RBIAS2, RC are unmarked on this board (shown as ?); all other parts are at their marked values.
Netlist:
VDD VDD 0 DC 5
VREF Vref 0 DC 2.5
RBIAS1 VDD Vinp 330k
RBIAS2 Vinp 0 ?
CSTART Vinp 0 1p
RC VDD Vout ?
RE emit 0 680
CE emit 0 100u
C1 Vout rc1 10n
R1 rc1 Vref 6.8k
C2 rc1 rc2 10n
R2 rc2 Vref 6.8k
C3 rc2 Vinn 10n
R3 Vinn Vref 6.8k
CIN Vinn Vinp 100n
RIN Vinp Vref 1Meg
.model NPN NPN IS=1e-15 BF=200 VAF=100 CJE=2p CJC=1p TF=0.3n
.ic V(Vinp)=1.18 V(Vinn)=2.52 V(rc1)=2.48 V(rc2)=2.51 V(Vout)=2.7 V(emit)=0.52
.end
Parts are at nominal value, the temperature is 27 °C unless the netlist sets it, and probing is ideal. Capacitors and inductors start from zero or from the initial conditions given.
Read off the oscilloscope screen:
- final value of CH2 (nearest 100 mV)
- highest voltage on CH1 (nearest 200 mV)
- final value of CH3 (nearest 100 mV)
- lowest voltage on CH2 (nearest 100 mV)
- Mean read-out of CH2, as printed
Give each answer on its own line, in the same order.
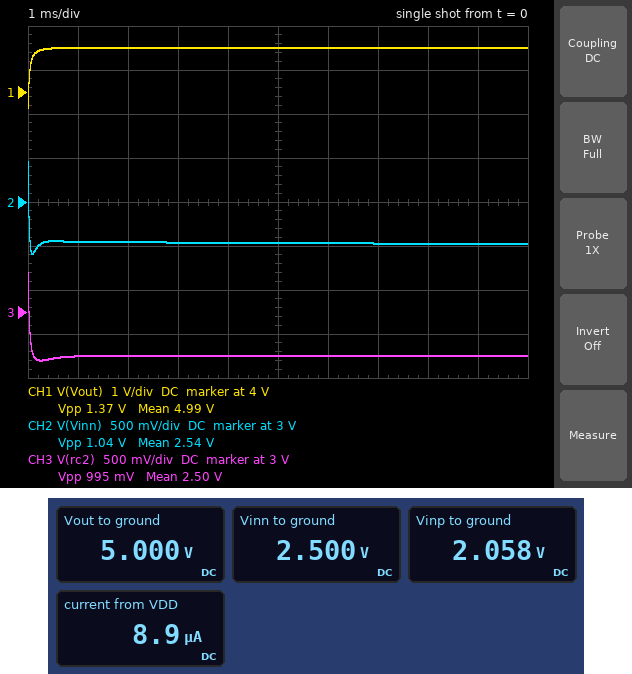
2.5 V
5.0 V
2.5 V
2.4 V
2.54 V
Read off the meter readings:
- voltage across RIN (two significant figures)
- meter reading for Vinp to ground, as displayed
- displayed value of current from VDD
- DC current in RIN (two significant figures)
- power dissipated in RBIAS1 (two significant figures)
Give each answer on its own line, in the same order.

440 mV
2.058 V
8.9 µA
440 nA
26 µW
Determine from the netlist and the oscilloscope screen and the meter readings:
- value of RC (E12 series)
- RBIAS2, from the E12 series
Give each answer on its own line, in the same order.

3.3 kΩ
220 kΩ
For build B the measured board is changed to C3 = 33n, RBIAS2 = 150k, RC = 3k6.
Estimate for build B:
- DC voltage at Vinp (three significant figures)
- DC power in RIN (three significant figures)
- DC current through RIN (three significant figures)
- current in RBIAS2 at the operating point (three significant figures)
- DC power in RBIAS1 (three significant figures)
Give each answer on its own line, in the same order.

1.65 V
722 nW
850 nA
11.0 µA
34.0 µW
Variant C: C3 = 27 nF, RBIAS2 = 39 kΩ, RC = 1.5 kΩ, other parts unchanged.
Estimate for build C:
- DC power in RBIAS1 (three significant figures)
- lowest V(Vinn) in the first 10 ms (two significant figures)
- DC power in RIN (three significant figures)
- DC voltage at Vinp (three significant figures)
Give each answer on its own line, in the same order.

58.8 µW
2.3 V
3.63 µW
595 mV
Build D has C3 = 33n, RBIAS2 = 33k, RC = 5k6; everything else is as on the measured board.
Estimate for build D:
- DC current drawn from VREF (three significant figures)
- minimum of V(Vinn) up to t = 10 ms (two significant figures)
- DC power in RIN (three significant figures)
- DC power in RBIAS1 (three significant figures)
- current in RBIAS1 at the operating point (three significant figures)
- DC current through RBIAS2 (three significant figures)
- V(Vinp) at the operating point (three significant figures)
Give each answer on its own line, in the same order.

1.99 µA
2.3 V
3.94 µW
61.0 µW
13.6 µA
15.6 µA
514 mV
